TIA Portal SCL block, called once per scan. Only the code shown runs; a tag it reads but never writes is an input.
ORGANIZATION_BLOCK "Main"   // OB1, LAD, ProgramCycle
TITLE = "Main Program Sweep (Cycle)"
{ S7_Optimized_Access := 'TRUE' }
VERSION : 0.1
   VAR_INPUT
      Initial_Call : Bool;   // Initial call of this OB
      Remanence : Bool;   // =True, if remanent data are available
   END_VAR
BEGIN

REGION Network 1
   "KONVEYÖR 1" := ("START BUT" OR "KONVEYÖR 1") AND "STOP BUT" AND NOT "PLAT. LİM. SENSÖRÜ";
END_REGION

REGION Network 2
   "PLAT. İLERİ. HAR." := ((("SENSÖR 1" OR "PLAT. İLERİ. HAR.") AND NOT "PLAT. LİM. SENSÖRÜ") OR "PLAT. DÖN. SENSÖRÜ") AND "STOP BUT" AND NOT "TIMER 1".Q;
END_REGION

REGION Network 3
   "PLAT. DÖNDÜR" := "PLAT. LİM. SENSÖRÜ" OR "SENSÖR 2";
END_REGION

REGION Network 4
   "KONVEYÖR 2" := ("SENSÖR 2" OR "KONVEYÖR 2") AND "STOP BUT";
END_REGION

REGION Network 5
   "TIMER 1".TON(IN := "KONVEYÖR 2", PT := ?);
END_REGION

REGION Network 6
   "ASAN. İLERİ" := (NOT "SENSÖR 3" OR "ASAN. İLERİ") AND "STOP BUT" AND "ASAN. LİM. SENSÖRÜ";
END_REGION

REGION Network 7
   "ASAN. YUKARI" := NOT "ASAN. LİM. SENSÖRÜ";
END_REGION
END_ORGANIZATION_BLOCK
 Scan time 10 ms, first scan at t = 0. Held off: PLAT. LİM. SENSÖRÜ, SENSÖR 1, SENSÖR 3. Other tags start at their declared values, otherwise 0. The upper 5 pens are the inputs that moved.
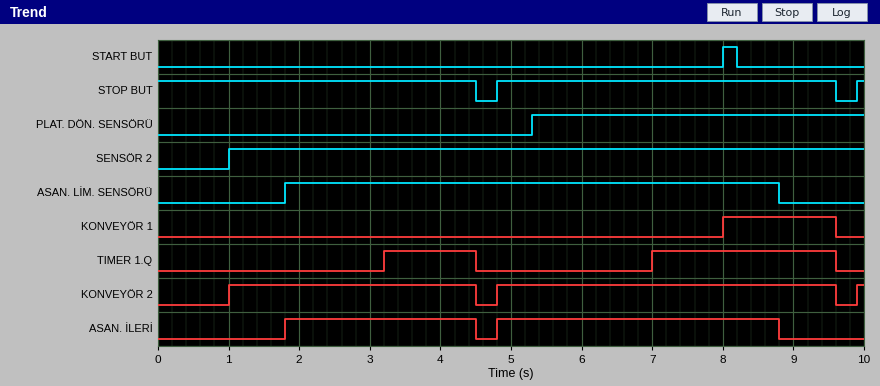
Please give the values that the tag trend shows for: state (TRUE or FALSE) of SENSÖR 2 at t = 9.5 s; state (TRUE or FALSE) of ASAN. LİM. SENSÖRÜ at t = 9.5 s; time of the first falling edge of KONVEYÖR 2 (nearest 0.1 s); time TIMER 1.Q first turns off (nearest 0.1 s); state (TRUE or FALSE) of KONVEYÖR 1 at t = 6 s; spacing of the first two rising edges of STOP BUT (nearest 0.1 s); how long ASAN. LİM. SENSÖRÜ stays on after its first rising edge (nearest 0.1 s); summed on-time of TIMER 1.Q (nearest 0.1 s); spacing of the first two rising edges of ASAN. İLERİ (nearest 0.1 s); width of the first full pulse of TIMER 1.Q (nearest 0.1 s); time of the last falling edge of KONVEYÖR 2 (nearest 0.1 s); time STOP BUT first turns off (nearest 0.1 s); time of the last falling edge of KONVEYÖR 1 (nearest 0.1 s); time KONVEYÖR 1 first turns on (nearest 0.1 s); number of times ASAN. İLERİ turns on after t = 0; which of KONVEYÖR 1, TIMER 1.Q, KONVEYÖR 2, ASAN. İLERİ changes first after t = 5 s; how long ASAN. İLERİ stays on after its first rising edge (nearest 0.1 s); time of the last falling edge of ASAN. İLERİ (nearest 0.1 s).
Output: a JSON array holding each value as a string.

["TRUE", "FALSE", "4.5 s", "4.5 s", "FALSE", "5.1 s", "7.0 s", "3.9 s", "3.0 s", "1.3 s", "9.6 s", "4.5 s", "9.6 s", "8.0 s", "2", "TIMER 1.Q", "2.7 s", "8.8 s"]
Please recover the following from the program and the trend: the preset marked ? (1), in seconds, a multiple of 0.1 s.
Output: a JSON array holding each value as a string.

["2.2 s"]
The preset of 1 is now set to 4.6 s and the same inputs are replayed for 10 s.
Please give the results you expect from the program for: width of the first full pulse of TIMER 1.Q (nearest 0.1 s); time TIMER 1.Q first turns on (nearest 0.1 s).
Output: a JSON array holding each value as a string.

["0.2 s", "9.4 s"]
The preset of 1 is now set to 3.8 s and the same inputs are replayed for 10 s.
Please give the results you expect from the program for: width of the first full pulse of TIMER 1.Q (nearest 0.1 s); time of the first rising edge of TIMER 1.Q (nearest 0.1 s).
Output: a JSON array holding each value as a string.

["1.0 s", "8.6 s"]
